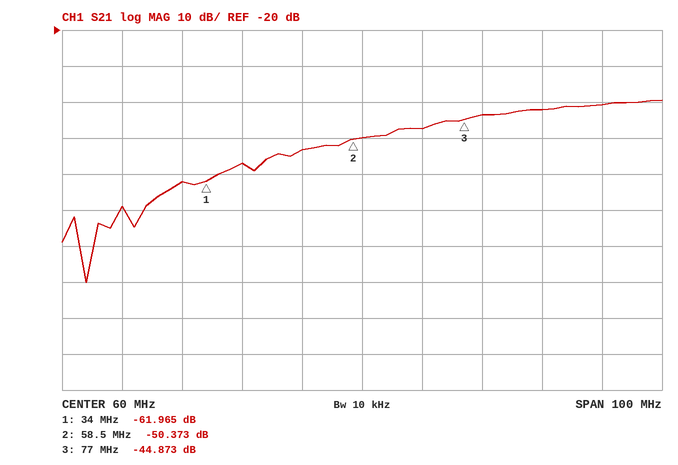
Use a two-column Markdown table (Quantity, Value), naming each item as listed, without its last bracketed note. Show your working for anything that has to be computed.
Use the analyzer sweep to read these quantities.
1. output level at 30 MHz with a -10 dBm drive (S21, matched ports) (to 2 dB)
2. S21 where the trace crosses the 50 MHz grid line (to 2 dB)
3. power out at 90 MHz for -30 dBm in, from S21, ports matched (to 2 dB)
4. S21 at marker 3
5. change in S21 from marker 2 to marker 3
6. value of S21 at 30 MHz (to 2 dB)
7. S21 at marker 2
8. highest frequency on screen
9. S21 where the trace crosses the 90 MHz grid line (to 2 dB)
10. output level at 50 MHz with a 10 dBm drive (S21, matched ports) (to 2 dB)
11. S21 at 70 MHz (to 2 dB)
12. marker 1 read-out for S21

| Quantity | Value |
|---|---|
| output level at 30 MHz with a -10 dBm drive (S21, matched ports) | -10 dBm + (-62 dB) = -72 dBm |
| S21 where the trace crosses the 50 MHz grid line | -54 dB |
| power out at 90 MHz for -30 dBm in, from S21, ports matched | -30 dBm + (-42 dB) = -72 dBm |
| S21 at marker 3 | -44.873 dB |
| change in S21 from marker 2 to marker 3 | -44.873 − (-50.373) = 5.500 dB |
| value of S21 at 30 MHz | -62 dB |
| S21 at marker 2 | -50.373 dB |
| highest frequency on screen | 110 MHz |
| S21 where the trace crosses the 90 MHz grid line | -42 dB |
| output level at 50 MHz with a 10 dBm drive (S21, matched ports) | 10 dBm + (-54 dB) = -44 dBm |
| S21 at 70 MHz | -48 dB |
| marker 1 read-out for S21 | -61.965 dB |
